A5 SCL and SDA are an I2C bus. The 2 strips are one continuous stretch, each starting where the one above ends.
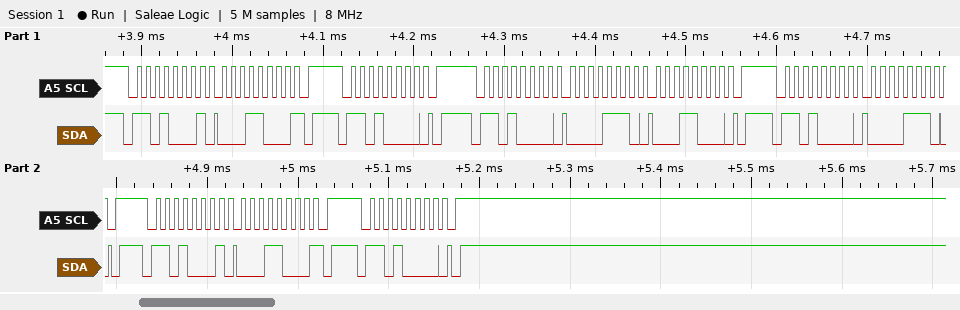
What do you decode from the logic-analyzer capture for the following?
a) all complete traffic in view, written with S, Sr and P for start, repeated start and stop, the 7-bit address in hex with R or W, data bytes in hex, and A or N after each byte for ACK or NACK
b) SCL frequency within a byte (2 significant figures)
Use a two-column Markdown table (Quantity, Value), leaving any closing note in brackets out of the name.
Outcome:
| Quantity | Value |
|---|---|
| all complete traffic in view, written with S, Sr and P for start, repeated start and stop, the 7-bit address in hex with R or W, data bytes in hex, and A or N after each byte for ACK or NACK | S 68R A 18 N P S 68W A P S 68W A 0E A 18 A P S 68W A 0E A P S 68R A 18 N P S 68W A P |
| SCL frequency within a byte | 100 kHz |
